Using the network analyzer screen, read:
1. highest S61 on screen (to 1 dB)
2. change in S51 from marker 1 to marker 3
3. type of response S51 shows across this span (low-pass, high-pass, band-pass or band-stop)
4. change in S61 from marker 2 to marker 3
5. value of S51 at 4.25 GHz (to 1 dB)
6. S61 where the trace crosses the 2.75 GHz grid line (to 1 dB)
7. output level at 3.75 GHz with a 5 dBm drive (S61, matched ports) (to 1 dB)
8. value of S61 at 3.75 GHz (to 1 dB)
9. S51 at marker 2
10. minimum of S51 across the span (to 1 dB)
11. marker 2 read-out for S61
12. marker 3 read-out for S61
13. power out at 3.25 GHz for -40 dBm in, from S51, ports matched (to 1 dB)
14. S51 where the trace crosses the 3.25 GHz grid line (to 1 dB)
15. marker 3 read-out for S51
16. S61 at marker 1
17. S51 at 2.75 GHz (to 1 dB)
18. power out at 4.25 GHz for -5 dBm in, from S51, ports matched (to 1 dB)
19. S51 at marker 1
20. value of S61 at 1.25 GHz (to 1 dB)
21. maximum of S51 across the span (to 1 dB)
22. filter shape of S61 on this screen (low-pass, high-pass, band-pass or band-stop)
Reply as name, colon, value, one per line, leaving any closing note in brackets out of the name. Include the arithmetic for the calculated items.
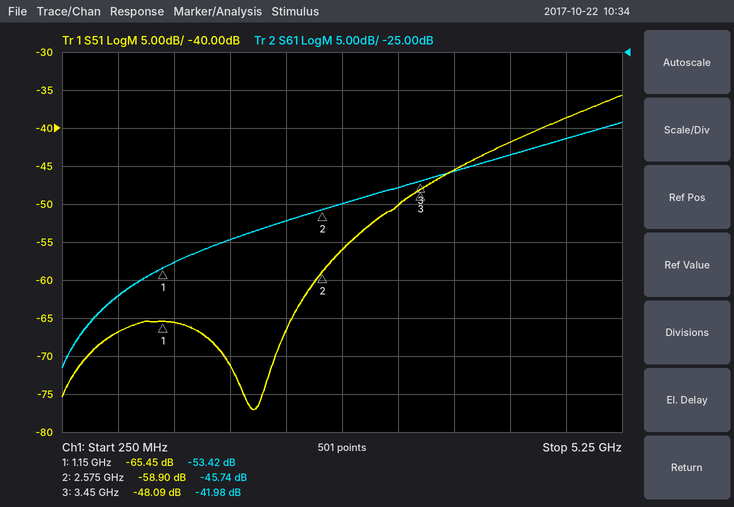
highest S61 on screen: -34 dB
change in S51 from marker 1 to marker 3: -48.09 − (-65.45) = 17.36 dB
type of response S51 shows across this span: high-pass
change in S61 from marker 2 to marker 3: -41.98 − (-45.74) = 3.76 dB
value of S51 at 4.25 GHz: -42 dB
S61 where the trace crosses the 2.75 GHz grid line: -45 dB
output level at 3.75 GHz with a 5 dBm drive (S61, matched ports): 5 dBm + (-41 dB) = -36 dBm
value of S61 at 3.75 GHz: -41 dB
S51 at marker 2: -58.90 dB
minimum of S51 across the span: -77 dB
marker 2 read-out for S61: -45.74 dB
marker 3 read-out for S61: -41.98 dB
power out at 3.25 GHz for -40 dBm in, from S51, ports matched: -40 dBm + (-50 dB) = -90 dBm
S51 where the trace crosses the 3.25 GHz grid line: -50 dB
marker 3 read-out for S51: -48.09 dB
S61 at marker 1: -53.42 dB
S51 at 2.75 GHz: -56 dB
power out at 4.25 GHz for -5 dBm in, from S51, ports matched: -5 dBm + (-42 dB) = -47 dBm
S51 at marker 1: -65.45 dB
value of S61 at 1.25 GHz: -53 dB
maximum of S51 across the span: -36 dB
filter shape of S61 on this screen: high-pass
